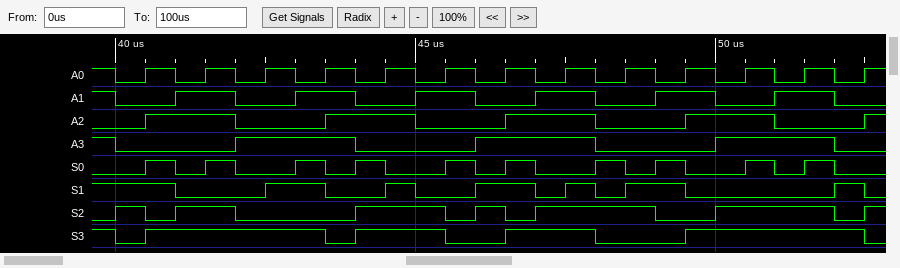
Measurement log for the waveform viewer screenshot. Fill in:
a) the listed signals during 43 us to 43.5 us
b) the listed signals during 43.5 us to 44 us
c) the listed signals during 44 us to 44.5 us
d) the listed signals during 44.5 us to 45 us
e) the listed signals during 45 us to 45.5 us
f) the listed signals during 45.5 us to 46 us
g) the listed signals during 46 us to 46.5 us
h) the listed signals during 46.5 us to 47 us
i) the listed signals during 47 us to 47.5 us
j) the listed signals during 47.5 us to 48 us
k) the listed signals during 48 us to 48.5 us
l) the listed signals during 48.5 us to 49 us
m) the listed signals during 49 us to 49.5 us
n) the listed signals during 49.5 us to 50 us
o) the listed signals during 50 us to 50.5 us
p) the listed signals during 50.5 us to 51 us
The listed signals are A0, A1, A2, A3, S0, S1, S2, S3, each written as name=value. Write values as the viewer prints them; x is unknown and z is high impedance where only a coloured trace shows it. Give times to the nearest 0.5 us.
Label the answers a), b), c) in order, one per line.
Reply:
a) A0=0, A1=1, A2=0, A3=1, S0=1, S1=1, S2=0, S3=1
b) A0=1, A1=1, A2=1, A3=1, S0=0, S1=0, S2=0, S3=0
c) A0=0, A1=0, A2=1, A3=0, S0=1, S1=0, S2=1, S3=1
d) A0=1, A1=0, A2=1, A3=0, S0=0, S1=1, S2=1, S3=1
e) A0=0, A1=1, A2=0, A3=0, S0=0, S1=0, S2=1, S3=1
f) A0=1, A1=1, A2=0, A3=0, S0=1, S1=0, S2=0, S3=0
g) A0=0, A1=0, A2=0, A3=1, S0=0, S1=1, S2=1, S3=0
h) A0=1, A1=0, A2=1, A3=1, S0=1, S1=1, S2=0, S3=1
i) A0=0, A1=1, A2=1, A3=1, S0=0, S1=0, S2=1, S3=1
j) A0=1, A1=1, A2=1, A3=1, S0=0, S1=1, S2=1, S3=1
k) A0=0, A1=0, A2=0, A3=0, S0=1, S1=0, S2=1, S3=0
l) A0=1, A1=0, A2=0, A3=0, S0=0, S1=1, S2=1, S3=0
m) A0=0, A1=1, A2=0, A3=0, S0=1, S1=1, S2=0, S3=0
n) A0=1, A1=1, A2=1, A3=0, S0=0, S1=0, S2=0, S3=1
o) A0=0, A1=0, A2=1, A3=1, S0=0, S1=0, S2=1, S3=1
p) A0=1, A1=0, A2=1, A3=1, S0=1, S1=0, S2=1, S3=1
